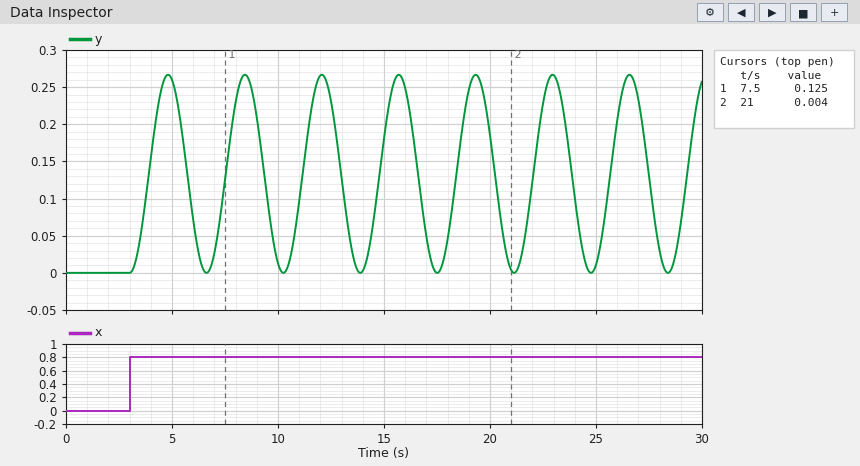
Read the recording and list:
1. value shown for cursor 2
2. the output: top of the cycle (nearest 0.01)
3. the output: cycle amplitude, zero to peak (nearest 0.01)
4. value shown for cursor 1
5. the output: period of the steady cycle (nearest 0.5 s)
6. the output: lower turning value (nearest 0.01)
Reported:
0.004
0.27
0.13
0.125
3.5 s
0.00
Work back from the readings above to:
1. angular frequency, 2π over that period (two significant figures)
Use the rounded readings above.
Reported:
1.8 rad/s
